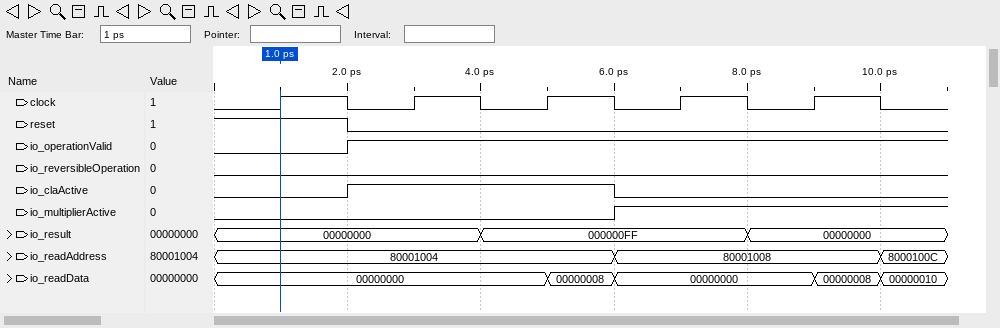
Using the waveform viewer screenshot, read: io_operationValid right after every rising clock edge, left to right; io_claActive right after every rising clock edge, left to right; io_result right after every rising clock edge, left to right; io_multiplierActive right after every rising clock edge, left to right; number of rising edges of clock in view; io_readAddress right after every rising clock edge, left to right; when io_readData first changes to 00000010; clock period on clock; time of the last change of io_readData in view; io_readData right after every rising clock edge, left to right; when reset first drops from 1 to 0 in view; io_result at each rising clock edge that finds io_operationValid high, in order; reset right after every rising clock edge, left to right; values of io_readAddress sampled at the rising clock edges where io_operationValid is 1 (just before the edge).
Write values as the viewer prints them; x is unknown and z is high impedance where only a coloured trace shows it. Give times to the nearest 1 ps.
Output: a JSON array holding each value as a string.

["0 1 1 1 1", "0 1 1 0 0", "00000000, 00000000, 000000FF, 000000FF, 00000000", "0 0 0 1 1", "5", "80001004, 80001004, 80001004, 80001008, 80001008", "10 ps", "2 ps", "10 ps", "00000000, 00000000, 00000008, 00000000, 00000008", "2 ps", "00000000, 000000FF, 000000FF, 00000000", "1 0 0 0 0", "80001004, 80001004, 80001008, 80001008"]
